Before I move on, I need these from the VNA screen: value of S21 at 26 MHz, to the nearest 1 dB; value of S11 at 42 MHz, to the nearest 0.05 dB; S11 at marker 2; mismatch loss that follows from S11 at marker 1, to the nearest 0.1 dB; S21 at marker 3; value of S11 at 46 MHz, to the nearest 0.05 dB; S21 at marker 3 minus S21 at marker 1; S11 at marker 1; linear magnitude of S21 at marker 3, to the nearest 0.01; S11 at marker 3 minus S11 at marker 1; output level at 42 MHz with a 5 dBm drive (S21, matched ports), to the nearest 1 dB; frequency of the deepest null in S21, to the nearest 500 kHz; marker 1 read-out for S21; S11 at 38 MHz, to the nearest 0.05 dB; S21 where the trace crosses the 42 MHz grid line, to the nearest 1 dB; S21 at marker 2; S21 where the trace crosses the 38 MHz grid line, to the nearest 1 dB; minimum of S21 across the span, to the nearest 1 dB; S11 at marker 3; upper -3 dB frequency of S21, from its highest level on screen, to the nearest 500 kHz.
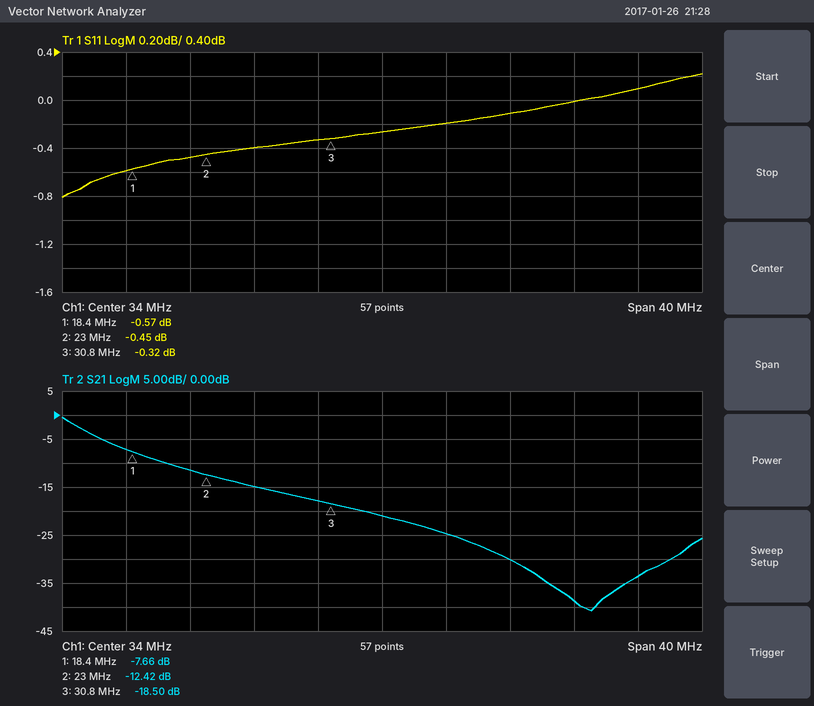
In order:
-15 dB
-0.10 dB
-0.45 dB
9.1 dB
-18.50 dB
0.00 dB
-10.84 dB
-0.57 dB
0.12
0.25 dB
-25 dBm
47.0 MHz
-7.66 dB
-0.20 dB
-30 dB
-12.42 dB
-25 dB
-41 dB
-0.32 dB
15.5 MHz
